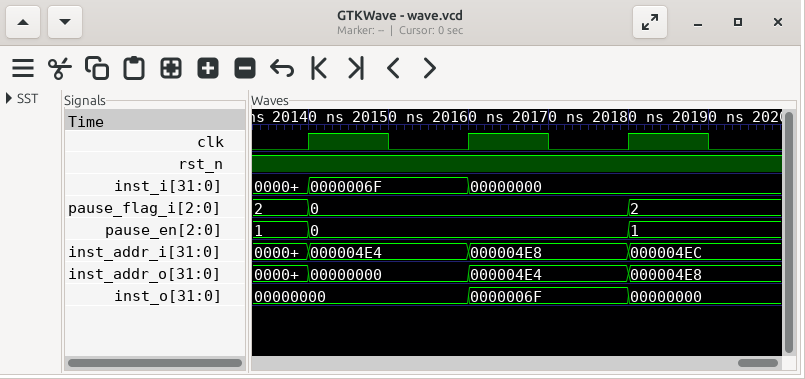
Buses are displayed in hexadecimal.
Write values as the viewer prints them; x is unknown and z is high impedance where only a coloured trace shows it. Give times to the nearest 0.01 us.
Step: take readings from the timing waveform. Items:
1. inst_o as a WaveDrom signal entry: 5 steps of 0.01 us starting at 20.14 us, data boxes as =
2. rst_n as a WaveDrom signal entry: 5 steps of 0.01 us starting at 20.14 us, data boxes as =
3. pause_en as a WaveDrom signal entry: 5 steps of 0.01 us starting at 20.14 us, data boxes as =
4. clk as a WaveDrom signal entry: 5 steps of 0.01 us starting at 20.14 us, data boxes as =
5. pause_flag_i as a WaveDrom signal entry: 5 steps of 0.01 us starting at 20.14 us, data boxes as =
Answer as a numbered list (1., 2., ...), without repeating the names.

1. {name: 'inst_o', wave: '=.=.=', data: '00000000 0000006F 00000000'}
2. {name: 'rst_n', wave: '1....'}
3. {name: 'pause_en', wave: '=...=', data: '0 1'}
4. {name: 'clk', wave: '10101'}
5. {name: 'pause_flag_i', wave: '=...=', data: '0 2'}
